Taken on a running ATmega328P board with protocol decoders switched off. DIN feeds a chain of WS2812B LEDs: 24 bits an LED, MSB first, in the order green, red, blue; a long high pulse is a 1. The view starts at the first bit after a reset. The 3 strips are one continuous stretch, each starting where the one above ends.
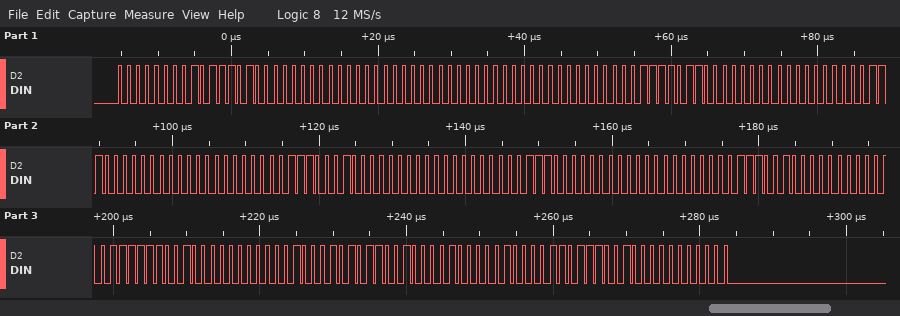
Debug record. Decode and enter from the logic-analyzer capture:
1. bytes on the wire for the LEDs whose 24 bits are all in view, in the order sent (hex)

00 BA 00 00 00 00 00 7B 00 00 38 00 00 71 00 00 1C 00 00 39 00 0F C8 00 8A C8 41 0D C8 00
